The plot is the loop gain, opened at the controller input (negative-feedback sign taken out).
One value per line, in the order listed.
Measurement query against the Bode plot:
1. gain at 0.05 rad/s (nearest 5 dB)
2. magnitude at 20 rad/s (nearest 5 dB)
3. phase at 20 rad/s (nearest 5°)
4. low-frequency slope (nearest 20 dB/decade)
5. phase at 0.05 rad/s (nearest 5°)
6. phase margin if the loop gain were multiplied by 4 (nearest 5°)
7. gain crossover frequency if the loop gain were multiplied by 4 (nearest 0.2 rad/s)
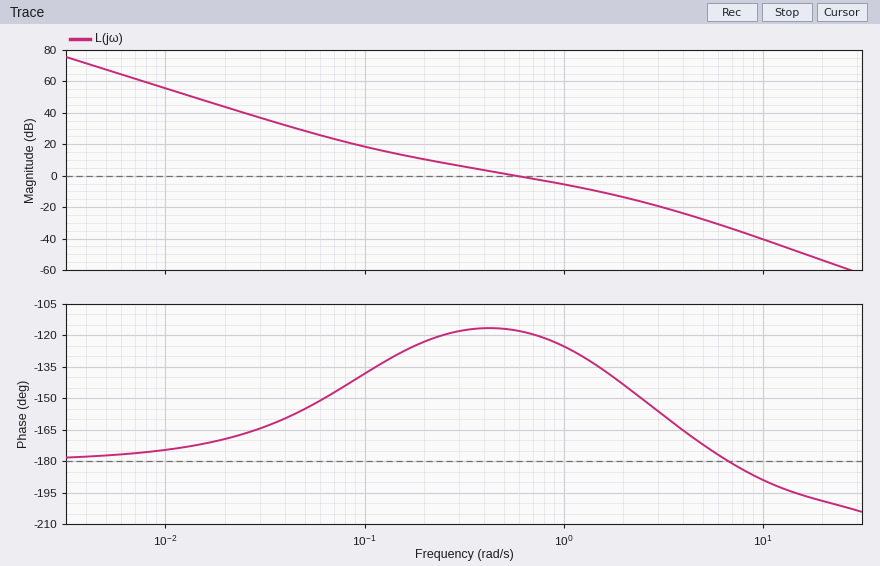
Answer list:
30 dB
-55 dB
-200°
-40 dB/decade
-155°
40°
1.8 rad/s
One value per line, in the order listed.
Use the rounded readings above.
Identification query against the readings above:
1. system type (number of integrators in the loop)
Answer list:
2
